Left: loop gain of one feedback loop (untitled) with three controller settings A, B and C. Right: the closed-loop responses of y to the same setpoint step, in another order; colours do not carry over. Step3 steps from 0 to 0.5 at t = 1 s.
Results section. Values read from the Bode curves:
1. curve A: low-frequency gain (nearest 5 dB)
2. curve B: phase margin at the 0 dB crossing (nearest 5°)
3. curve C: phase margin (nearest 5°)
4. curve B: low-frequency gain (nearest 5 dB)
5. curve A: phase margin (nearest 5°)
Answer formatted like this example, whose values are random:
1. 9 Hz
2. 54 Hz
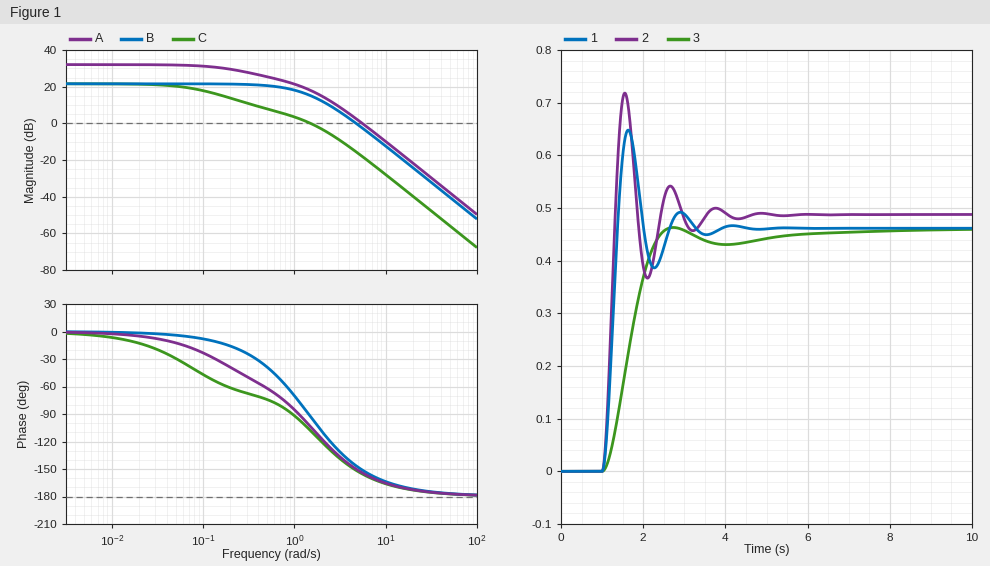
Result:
1. 30 dB
2. 35°
3. 70°
4. 20 dB
5. 25°
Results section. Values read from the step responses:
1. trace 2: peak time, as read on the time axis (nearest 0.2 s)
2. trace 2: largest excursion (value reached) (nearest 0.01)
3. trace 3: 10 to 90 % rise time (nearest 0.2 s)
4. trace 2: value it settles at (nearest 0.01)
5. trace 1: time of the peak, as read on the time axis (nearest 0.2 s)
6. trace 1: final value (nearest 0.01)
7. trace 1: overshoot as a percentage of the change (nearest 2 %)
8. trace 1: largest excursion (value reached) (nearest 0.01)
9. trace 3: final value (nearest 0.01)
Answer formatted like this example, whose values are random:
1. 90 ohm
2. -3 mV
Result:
1. 1.6 s
2. 0.72
3. 1.0 s
4. 0.49
5. 1.6 s
6. 0.46
7. 40 %
8. 0.65
9. 0.46
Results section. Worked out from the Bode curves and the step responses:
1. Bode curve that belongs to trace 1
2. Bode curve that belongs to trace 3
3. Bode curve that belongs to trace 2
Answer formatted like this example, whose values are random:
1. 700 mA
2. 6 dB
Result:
1. B
2. C
3. A
